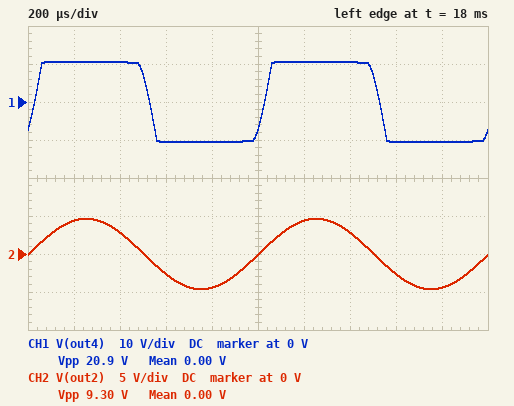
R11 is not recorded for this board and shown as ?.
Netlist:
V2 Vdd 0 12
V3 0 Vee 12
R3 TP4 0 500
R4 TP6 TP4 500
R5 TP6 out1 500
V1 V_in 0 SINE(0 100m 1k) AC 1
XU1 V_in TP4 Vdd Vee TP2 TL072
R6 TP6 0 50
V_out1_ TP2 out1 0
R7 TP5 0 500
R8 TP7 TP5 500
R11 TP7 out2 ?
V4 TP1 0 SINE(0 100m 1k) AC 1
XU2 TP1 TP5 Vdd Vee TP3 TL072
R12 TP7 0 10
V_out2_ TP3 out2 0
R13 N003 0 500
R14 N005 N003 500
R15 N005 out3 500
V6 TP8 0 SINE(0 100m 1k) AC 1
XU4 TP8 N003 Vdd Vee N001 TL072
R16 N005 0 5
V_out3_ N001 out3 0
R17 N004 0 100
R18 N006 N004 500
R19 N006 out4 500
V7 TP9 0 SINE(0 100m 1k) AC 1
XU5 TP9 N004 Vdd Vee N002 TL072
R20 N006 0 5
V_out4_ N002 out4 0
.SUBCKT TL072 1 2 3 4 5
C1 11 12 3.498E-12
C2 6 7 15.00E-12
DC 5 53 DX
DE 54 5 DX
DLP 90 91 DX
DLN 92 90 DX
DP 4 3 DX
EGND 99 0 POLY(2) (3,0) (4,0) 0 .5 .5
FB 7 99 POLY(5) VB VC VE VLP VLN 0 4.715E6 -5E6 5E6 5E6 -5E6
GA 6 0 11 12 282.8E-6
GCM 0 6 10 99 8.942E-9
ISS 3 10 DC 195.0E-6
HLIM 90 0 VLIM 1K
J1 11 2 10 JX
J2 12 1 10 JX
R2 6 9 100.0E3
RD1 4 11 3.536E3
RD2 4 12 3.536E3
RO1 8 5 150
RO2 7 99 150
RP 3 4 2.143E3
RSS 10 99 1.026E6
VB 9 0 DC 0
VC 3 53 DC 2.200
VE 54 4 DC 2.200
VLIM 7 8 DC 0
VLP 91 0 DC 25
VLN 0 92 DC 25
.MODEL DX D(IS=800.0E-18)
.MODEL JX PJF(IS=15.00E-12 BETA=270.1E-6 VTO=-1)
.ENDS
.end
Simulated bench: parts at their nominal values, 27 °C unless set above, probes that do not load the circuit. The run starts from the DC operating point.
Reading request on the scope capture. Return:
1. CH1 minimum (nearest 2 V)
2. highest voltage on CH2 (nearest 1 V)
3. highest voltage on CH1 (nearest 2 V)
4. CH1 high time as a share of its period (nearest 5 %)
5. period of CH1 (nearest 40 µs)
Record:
-10 V
5 V
10 V
50 %
1.00 ms
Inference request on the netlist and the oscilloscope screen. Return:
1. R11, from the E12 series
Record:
220 Ω
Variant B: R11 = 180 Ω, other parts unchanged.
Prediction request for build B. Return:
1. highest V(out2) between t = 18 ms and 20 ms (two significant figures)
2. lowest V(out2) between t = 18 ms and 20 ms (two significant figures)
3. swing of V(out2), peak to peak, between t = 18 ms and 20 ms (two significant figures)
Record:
3.8 V
-3.8 V
7.7 V
